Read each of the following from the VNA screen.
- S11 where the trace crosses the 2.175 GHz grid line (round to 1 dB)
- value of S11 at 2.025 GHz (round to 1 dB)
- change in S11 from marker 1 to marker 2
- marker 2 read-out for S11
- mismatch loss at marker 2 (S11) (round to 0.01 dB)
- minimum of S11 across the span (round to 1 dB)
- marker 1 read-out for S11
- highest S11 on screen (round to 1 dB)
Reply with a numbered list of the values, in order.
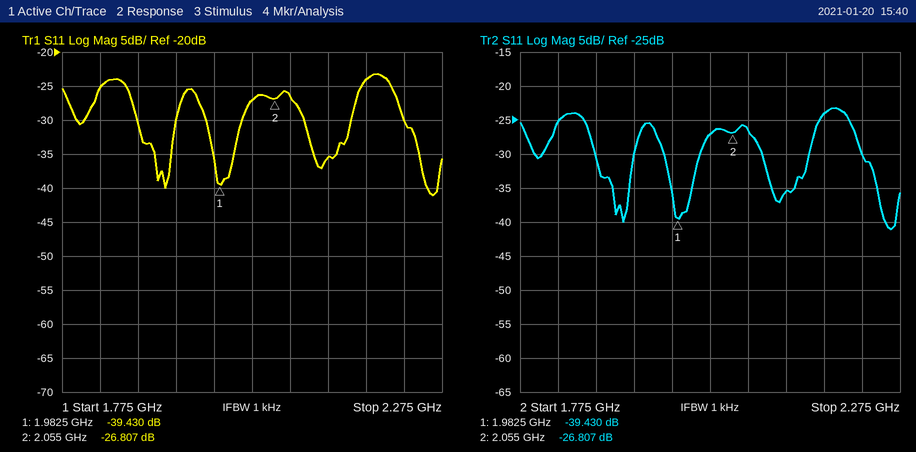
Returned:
1. -24 dB
2. -27 dB
3. 12.623 dB
4. -26.807 dB
5. 0.01 dB
6. -41 dB
7. -39.430 dB
8. -23 dB
